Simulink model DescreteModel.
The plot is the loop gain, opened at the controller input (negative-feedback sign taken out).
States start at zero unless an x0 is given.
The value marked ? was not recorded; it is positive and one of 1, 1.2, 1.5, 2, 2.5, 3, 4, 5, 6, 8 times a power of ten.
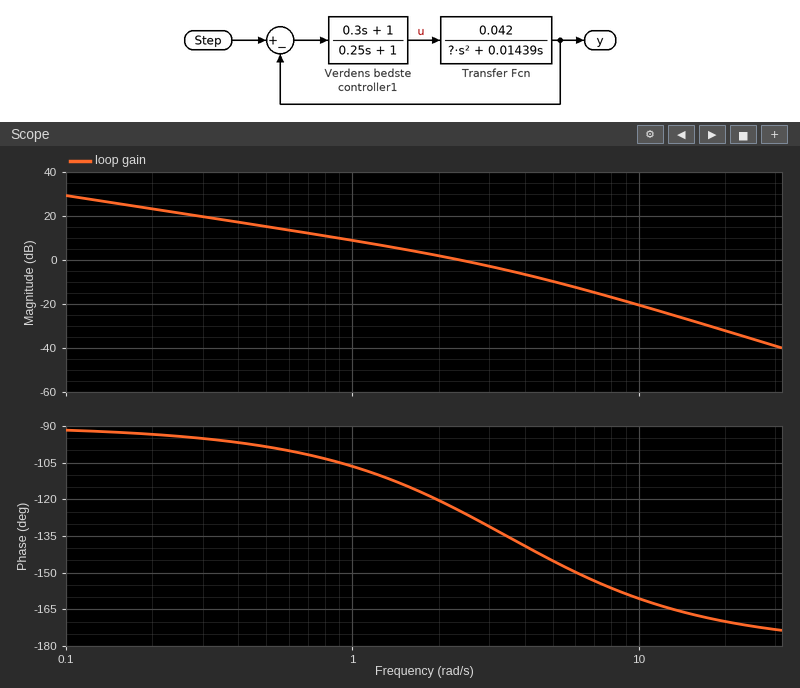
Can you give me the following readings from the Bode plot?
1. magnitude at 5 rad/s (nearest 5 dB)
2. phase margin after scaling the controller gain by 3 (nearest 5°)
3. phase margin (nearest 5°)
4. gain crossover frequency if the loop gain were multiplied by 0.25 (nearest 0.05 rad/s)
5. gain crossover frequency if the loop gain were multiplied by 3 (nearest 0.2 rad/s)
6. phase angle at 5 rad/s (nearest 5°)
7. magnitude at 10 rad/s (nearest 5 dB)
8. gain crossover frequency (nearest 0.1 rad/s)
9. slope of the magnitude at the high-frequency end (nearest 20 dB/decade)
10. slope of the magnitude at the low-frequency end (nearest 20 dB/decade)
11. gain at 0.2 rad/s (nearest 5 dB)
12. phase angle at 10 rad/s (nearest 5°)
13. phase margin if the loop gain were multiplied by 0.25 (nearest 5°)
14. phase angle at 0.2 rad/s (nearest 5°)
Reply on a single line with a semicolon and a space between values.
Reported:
-10 dB; 35°; 55°; 0.70 rad/s; 5.0 rad/s; -145°; -20 dB; 2.4 rad/s; -40 dB/decade; -20 dB/decade; 25 dB; -160°; 80°; -95°
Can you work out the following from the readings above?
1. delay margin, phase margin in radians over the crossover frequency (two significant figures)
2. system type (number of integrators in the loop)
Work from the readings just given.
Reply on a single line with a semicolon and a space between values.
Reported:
0.40 s; 1
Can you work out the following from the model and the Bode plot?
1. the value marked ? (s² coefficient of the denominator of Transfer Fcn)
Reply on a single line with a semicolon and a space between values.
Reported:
0.005
